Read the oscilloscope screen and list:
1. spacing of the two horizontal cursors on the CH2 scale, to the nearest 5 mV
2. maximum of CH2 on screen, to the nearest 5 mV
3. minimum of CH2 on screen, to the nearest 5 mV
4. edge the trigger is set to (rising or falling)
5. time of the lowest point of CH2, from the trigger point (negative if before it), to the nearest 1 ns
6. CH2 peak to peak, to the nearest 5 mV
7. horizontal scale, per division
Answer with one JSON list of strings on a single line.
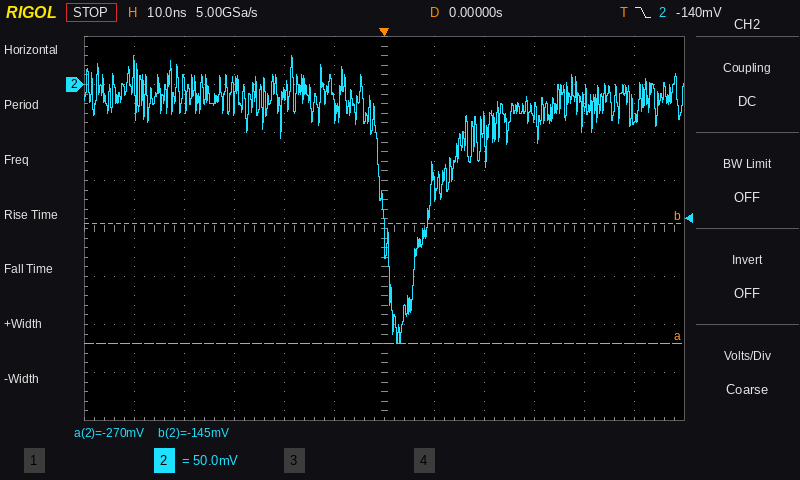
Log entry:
["125 mV", "30 mV", "-270 mV", "falling", "+3 ns", "300 mV", "10 ns"]
